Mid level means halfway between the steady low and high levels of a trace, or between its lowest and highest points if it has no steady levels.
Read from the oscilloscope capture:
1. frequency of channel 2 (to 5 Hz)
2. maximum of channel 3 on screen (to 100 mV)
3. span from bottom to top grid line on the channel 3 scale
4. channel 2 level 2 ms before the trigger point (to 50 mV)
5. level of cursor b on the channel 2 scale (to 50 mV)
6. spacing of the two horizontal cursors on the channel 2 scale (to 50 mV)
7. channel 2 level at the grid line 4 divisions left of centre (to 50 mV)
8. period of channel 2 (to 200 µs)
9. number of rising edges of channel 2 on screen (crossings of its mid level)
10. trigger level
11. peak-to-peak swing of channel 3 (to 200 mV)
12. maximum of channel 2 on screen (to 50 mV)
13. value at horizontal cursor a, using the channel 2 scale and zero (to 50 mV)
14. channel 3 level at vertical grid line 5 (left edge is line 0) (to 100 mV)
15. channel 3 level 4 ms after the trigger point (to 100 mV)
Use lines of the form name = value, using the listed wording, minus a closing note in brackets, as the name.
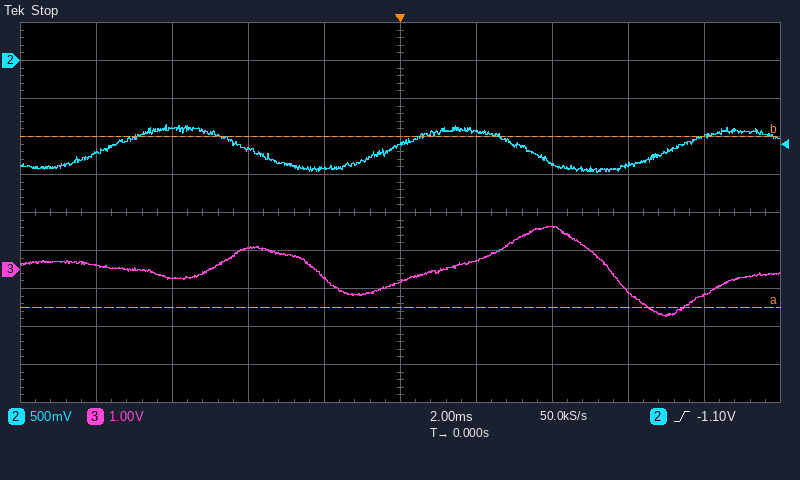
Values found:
frequency of channel 2 = 135 Hz
maximum of channel 3 on screen = 1.1 V
span from bottom to top grid line on the channel 3 scale = 10 V
channel 2 level 2 ms before the trigger point = -1.40 V
level of cursor b on the channel 2 scale = -1.00 V
spacing of the two horizontal cursors on the channel 2 scale = 2.25 V
channel 2 level at the grid line 4 divisions left of centre = -1.20 V
period of channel 2 = 7.4 ms
number of rising edges of channel 2 on screen = 3
trigger level = -1.10 V
peak-to-peak swing of channel 3 = 2.4 V
maximum of channel 2 on screen = -850 mV
value at horizontal cursor a, using the channel 2 scale and zero = -3.25 V
channel 3 level at vertical grid line 5 (left edge is line 0) = -300 mV
channel 3 level 4 ms after the trigger point = 1.1 V
